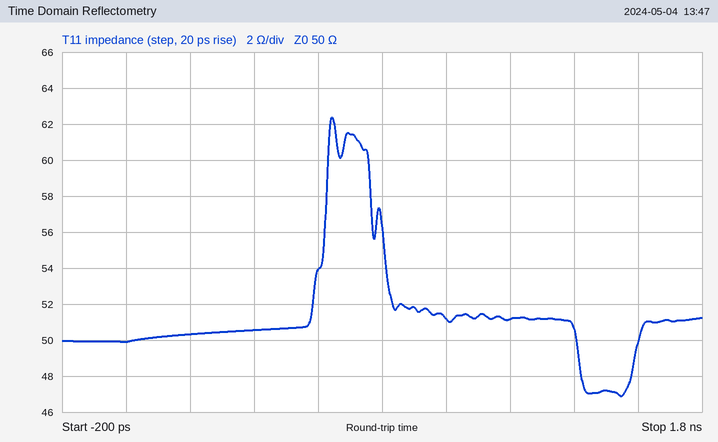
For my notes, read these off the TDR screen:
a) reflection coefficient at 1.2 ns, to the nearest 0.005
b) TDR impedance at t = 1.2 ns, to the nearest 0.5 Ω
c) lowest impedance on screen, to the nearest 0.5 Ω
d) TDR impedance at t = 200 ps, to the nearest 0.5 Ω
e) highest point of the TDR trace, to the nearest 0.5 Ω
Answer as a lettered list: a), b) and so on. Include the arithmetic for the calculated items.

a) (51 − 50)/(51 + 50) ≈ +0.010
b) 51.0 Ω
c) 47.0 Ω
d) 50.5 Ω
e) 62.5 Ω
